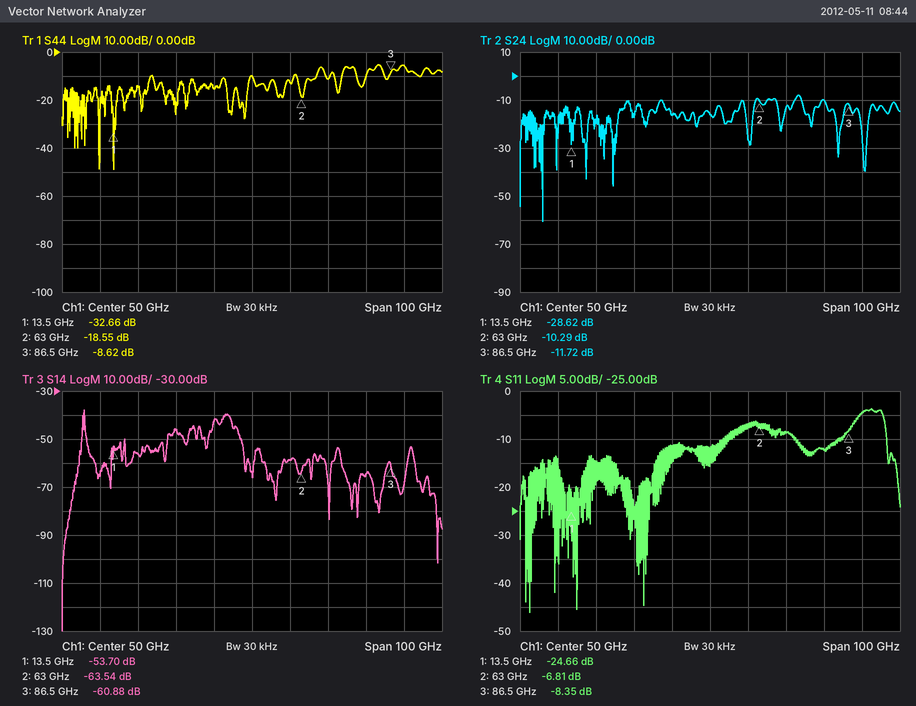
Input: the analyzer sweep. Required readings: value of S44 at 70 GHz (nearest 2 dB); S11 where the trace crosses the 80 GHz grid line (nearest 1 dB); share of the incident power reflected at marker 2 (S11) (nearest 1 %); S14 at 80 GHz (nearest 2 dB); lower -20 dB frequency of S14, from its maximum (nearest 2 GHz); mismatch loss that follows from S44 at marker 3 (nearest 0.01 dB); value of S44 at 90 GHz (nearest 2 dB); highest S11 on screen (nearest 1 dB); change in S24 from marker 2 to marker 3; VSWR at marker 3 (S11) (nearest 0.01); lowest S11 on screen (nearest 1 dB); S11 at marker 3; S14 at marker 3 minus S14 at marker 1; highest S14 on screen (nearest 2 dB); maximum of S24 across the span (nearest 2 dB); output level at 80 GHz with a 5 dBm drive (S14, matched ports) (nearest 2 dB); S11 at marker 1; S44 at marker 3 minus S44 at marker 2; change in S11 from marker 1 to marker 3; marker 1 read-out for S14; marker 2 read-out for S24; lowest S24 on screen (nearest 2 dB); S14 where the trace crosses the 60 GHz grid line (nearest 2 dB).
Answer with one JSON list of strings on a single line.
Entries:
["-12 dB", "-12 dB", "21 %", "-64 dB", "4 GHz", "0.64 dB", "-6 dB", "-4 dB", "-1.43 dB", "2.24", "-46 dB", "-8.35 dB", "-7.18 dB", "-38 dB", "-8 dB", "-60 dBm", "-24.66 dB", "9.93 dB", "16.31 dB", "-53.70 dB", "-10.29 dB", "-60 dB", "-58 dB"]
